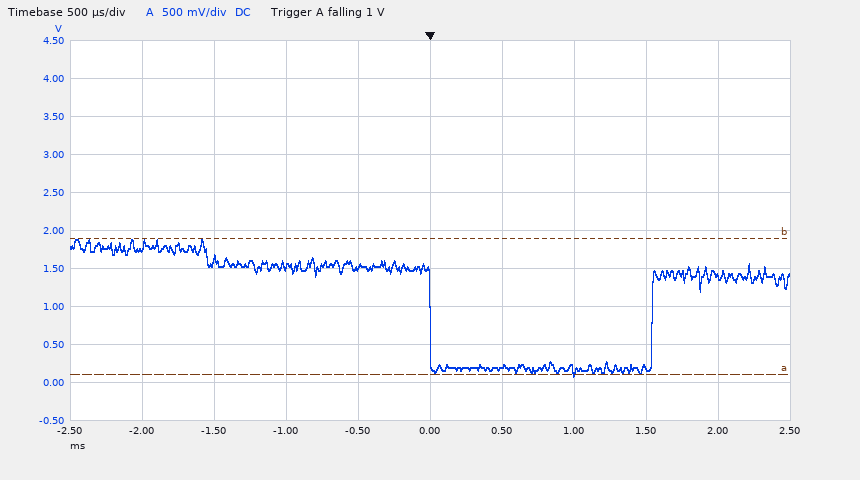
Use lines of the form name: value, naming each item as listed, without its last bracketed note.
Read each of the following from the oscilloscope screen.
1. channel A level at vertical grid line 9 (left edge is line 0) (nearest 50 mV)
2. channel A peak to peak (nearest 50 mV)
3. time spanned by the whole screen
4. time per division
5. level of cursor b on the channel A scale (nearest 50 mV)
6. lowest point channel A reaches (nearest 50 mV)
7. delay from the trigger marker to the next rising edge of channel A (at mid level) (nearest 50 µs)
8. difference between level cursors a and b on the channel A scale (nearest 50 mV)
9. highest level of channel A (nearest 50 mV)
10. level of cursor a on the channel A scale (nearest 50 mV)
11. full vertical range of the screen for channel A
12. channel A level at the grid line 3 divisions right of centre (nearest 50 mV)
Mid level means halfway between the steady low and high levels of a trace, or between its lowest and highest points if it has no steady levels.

channel A level at vertical grid line 9 (left edge is line 0): 1.40 V
channel A peak to peak: 1.80 V
time spanned by the whole screen: 5 ms
time per division: 500 µs
level of cursor b on the channel A scale: 1.90 V
lowest point channel A reaches: 100 mV
delay from the trigger marker to the next rising edge of channel A (at mid level): 1.55 ms
difference between level cursors a and b on the channel A scale: 1.80 V
highest level of channel A: 1.90 V
level of cursor a on the channel A scale: 100 mV
full vertical range of the screen for channel A: 5 V
channel A level at the grid line 3 divisions right of centre: 200 mV
